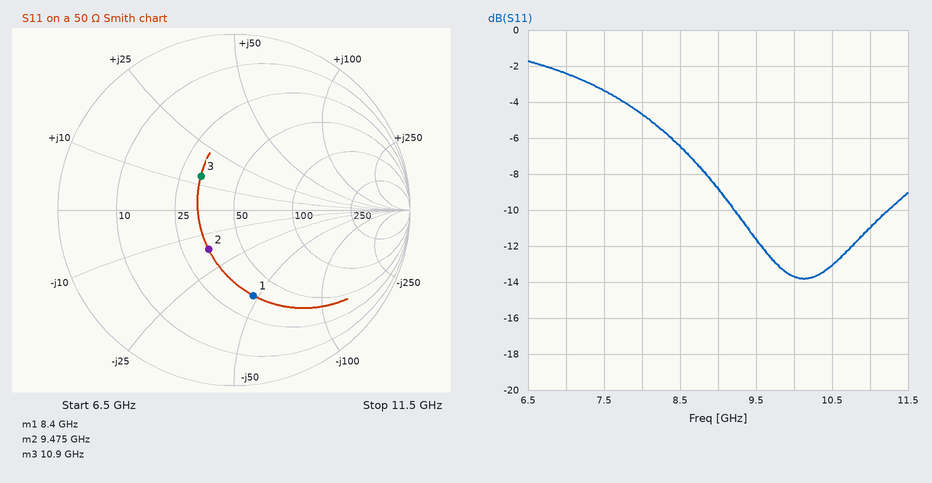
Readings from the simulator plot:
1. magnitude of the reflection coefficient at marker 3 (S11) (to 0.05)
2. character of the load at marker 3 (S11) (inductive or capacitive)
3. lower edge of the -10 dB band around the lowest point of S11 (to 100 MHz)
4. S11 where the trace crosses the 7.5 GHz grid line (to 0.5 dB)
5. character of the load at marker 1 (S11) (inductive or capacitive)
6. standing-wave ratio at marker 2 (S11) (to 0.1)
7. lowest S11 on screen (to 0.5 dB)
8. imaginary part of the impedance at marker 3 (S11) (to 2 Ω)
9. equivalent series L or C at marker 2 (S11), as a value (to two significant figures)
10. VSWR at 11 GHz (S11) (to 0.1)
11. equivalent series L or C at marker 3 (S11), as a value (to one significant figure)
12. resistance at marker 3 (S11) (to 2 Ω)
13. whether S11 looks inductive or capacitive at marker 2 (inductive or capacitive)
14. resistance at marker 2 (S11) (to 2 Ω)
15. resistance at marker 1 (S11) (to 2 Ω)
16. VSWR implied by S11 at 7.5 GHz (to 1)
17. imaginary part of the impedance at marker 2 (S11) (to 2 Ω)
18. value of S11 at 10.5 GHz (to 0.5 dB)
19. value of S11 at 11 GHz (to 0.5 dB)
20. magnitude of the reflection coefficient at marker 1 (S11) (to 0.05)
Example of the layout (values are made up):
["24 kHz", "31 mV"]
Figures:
["0.25", "inductive", "9.2 GHz", "-3.5 dB", "capacitive", "1.7", "-14.0 dB", "+14 Ω", "1.0 pF", "1.8", "200 pH", "32 Ω", "capacitive", "34 Ω", "36 Ω", "5", "-16 Ω", "-13.0 dB", "-11.0 dB", "0.50"]
